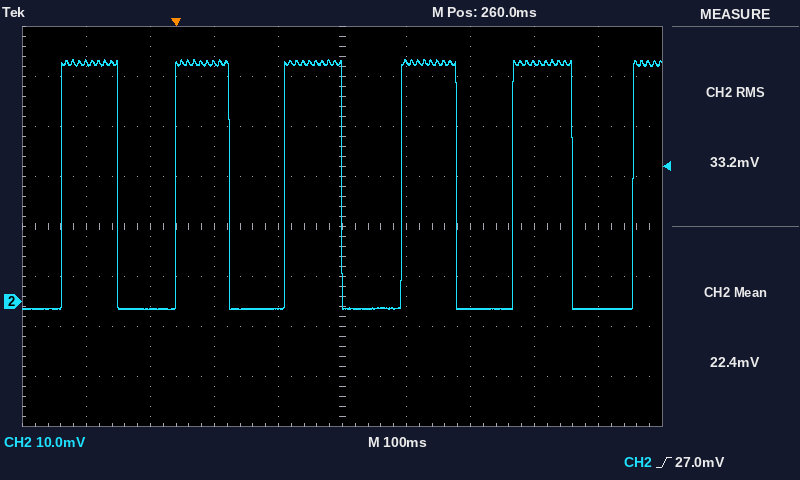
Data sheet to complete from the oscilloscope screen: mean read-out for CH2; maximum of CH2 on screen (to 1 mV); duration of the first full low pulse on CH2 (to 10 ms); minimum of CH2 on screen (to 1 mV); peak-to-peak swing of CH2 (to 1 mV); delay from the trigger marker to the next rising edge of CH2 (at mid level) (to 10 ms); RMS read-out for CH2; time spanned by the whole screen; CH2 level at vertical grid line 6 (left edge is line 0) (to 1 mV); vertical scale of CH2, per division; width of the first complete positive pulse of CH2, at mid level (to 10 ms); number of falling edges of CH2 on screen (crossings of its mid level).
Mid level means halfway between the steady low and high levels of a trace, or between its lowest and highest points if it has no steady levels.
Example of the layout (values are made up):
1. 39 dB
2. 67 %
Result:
1. 22.4 mV
2. 48 mV
3. 90 ms
4. -2 mV
5. 50 mV
6. 170 ms
7. 33.2 mV
8. 1 s
9. 48 mV
10. 10 mV
11. 90 ms
12. 5
